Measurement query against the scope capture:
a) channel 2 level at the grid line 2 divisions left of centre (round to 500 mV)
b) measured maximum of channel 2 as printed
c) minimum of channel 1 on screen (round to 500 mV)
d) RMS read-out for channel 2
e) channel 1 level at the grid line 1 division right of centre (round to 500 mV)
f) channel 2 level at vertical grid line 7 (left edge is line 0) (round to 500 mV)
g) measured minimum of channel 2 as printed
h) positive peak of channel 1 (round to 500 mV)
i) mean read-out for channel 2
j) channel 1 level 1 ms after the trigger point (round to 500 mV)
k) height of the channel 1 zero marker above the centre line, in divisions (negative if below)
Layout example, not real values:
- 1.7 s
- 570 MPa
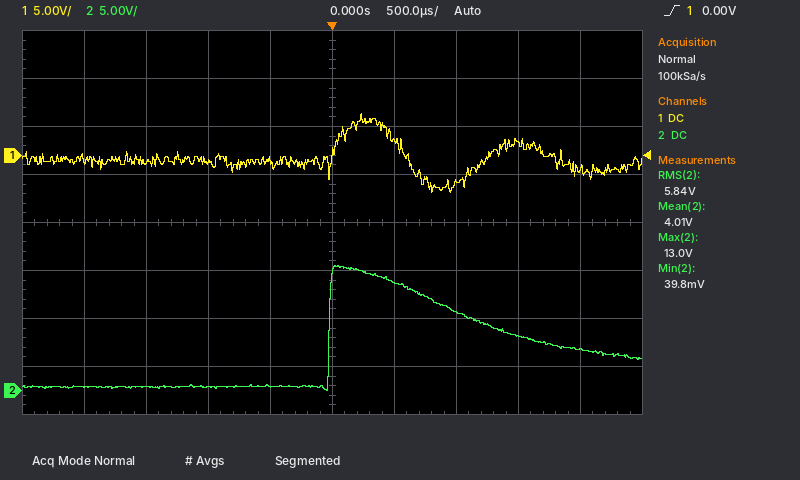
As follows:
- 500 mV
- 13.0 V
- -4.0 V
- 5.84 V
- 1.5 V
- 8.0 V
- 39.8 mV
- 4.5 V
- 4.01 V
- -3.0 V
- +1.4 div
